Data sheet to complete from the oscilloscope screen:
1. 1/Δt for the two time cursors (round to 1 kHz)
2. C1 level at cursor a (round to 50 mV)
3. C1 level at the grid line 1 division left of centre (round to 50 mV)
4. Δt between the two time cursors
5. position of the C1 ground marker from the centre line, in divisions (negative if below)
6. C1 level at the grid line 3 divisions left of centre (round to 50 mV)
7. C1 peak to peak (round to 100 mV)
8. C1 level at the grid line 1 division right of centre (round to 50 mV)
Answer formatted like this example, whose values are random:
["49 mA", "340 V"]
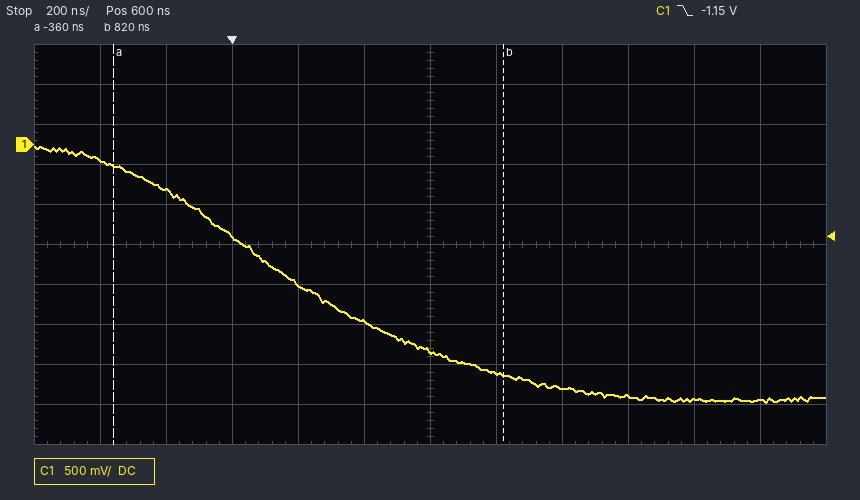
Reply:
["847 kHz", "-250 mV", "-2.20 V", "1.18 µs", "+2.5 div", "-1.15 V", "3.20 V", "-2.85 V"]
